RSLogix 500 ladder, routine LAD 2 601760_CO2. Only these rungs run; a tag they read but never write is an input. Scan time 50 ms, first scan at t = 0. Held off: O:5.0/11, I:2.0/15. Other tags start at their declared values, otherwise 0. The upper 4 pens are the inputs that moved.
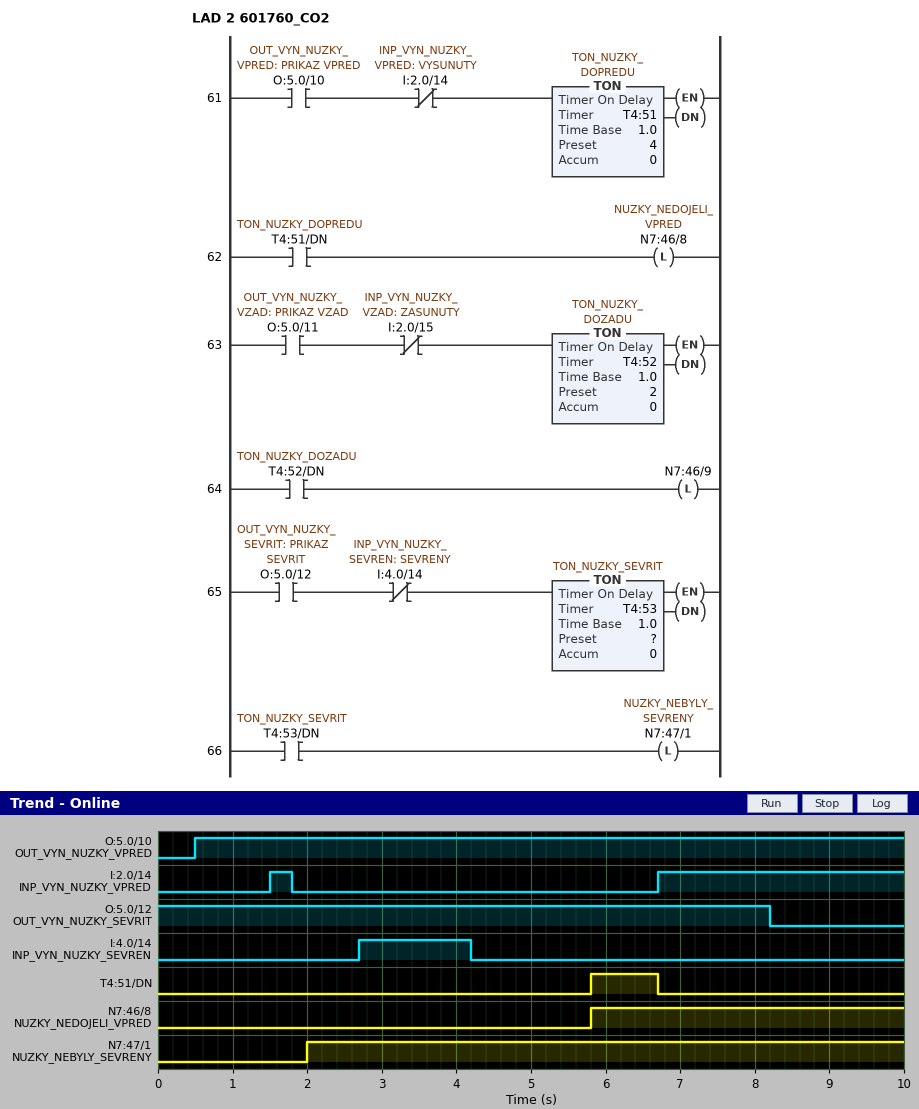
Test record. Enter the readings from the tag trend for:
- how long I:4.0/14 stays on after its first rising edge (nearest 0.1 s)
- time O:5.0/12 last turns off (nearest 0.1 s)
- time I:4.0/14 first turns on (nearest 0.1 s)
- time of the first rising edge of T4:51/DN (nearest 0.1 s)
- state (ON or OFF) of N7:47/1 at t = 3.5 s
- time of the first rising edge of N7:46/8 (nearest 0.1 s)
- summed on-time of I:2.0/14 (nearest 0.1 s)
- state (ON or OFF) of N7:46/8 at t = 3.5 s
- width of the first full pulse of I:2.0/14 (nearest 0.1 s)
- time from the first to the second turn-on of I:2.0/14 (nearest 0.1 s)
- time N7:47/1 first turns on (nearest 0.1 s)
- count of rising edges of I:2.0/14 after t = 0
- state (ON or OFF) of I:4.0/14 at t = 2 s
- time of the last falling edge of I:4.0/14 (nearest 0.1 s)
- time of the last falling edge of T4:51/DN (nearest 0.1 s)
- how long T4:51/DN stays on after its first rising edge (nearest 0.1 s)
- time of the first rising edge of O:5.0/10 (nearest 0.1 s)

1.5 s
8.2 s
2.7 s
5.8 s
ON
5.8 s
3.6 s
OFF
0.3 s
5.2 s
2.0 s
2
OFF
4.2 s
6.7 s
0.9 s
0.5 s
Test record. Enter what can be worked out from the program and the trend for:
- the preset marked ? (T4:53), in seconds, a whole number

2 s
